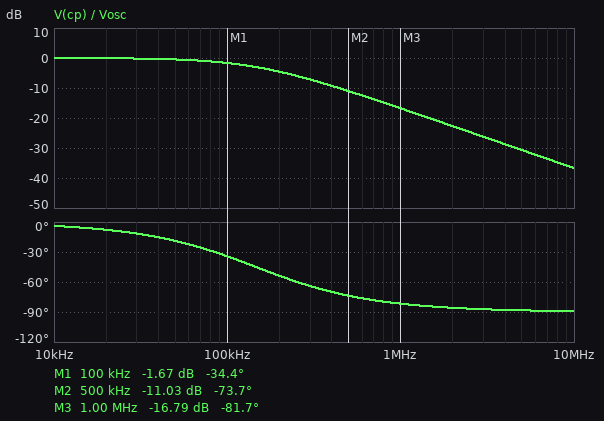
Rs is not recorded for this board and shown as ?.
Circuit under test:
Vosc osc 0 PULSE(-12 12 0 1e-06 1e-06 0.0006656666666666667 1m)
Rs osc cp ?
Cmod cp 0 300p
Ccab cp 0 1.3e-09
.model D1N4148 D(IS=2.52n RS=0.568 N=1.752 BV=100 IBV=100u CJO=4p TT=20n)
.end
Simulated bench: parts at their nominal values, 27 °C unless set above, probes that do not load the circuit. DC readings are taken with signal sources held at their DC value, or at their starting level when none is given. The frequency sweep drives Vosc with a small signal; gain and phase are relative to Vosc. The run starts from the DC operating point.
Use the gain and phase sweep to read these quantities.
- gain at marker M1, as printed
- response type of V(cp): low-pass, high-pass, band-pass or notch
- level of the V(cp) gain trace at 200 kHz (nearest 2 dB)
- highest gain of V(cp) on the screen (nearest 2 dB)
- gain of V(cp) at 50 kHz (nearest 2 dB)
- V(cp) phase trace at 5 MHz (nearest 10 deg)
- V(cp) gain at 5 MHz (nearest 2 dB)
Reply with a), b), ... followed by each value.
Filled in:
a) -1.67 dB
b) low-pass
c) -4 dB
d) 0 dB
e) 0 dB
f) -90 deg
g) -30 dB
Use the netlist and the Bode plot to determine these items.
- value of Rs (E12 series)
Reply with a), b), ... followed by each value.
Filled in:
a) 680 Ω
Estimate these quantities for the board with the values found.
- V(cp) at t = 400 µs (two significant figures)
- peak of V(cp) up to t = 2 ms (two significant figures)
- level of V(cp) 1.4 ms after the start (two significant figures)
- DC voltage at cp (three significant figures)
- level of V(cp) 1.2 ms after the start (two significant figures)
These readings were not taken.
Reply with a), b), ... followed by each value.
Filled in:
a) 12 V
b) 12 V
c) 12 V
d) -12.0 V
e) 12 V
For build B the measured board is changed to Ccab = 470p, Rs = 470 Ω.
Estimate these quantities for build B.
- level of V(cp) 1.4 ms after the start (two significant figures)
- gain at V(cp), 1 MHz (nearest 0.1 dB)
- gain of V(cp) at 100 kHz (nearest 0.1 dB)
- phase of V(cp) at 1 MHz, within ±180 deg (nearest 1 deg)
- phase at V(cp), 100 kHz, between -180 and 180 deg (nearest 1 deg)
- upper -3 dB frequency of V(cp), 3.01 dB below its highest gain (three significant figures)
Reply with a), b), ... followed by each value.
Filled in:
a) 12 V
b) -7.9 dB
c) -0.2 dB
d) -66 deg
e) -13 deg
f) 440 kHz
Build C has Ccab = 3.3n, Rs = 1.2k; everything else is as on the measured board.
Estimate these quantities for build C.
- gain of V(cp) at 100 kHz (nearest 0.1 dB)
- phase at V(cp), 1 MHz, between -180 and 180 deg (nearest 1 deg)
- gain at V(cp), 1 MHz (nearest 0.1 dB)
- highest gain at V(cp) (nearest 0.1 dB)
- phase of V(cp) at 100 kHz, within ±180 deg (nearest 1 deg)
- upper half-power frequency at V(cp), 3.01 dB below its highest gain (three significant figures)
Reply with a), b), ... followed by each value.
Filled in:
a) -9.2 dB
b) -88 deg
c) -28.7 dB
d) 0 dB
e) -70 deg
f) 36.8 kHz
